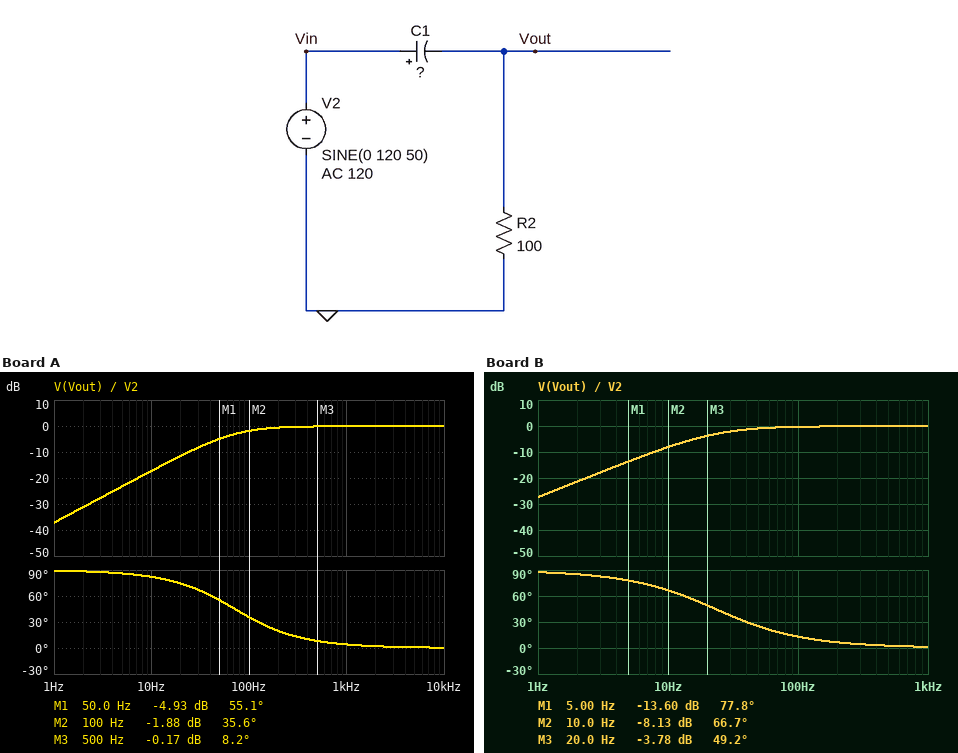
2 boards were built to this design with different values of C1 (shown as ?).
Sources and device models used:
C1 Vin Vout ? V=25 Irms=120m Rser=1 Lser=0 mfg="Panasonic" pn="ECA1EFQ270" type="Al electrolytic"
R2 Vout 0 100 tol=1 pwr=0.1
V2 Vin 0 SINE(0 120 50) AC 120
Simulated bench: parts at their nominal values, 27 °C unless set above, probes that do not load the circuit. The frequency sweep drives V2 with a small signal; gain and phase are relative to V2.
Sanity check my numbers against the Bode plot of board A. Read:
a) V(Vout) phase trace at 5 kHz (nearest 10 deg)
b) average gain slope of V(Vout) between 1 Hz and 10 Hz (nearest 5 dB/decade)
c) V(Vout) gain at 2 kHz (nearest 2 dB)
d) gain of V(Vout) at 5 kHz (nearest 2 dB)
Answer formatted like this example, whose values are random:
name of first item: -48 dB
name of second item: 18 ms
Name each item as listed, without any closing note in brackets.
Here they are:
V(Vout) phase trace at 5 kHz: 0 deg
average gain slope of V(Vout) between 1 Hz and 10 Hz: 20 dB/decade
V(Vout) gain at 2 kHz: 0 dB
gain of V(Vout) at 5 kHz: 0 dB
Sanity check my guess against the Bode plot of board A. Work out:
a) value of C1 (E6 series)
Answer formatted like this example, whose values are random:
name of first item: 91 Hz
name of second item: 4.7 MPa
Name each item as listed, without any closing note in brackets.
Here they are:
value of C1: 22 µF
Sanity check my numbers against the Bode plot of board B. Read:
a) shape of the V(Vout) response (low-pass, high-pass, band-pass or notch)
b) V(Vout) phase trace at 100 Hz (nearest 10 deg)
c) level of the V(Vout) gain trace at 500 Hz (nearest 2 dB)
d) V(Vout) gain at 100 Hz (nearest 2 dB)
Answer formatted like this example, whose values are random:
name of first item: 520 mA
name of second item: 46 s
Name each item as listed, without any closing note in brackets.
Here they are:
shape of the V(Vout) response: high-pass
V(Vout) phase trace at 100 Hz: 10 deg
level of the V(Vout) gain trace at 500 Hz: 0 dB
V(Vout) gain at 100 Hz: 0 dB
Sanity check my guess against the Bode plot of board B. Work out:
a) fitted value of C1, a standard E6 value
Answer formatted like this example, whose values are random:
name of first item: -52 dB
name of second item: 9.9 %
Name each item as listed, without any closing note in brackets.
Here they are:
fitted value of C1, a standard E6 value: 68 µF
